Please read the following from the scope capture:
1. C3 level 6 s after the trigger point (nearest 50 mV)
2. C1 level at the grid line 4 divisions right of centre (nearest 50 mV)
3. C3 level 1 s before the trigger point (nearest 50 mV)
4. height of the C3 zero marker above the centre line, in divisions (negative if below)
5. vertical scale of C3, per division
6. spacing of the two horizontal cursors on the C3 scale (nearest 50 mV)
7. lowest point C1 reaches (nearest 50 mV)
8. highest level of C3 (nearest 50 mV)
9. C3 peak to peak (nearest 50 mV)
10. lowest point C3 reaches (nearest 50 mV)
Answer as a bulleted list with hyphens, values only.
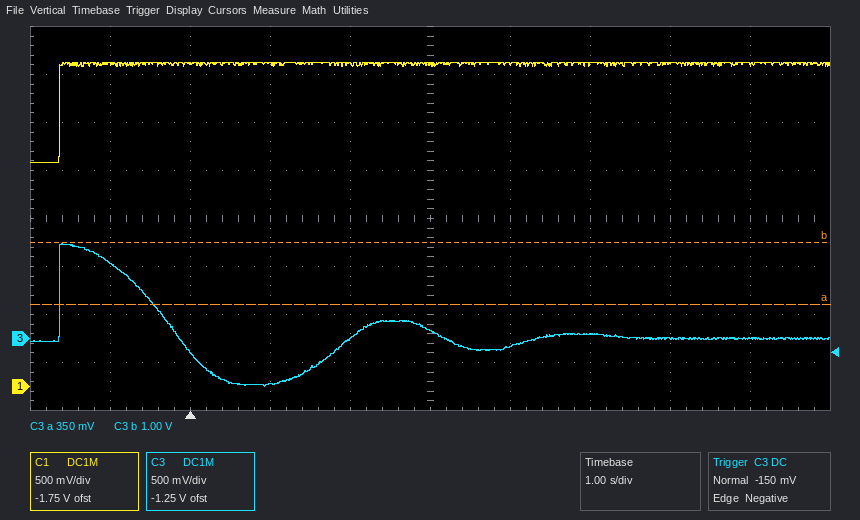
- 0 mV
- 3.35 V
- 800 mV
- -2.5 div
- 500 mV
- 650 mV
- 2.35 V
- 1.00 V
- 1.50 V
- -500 mV
